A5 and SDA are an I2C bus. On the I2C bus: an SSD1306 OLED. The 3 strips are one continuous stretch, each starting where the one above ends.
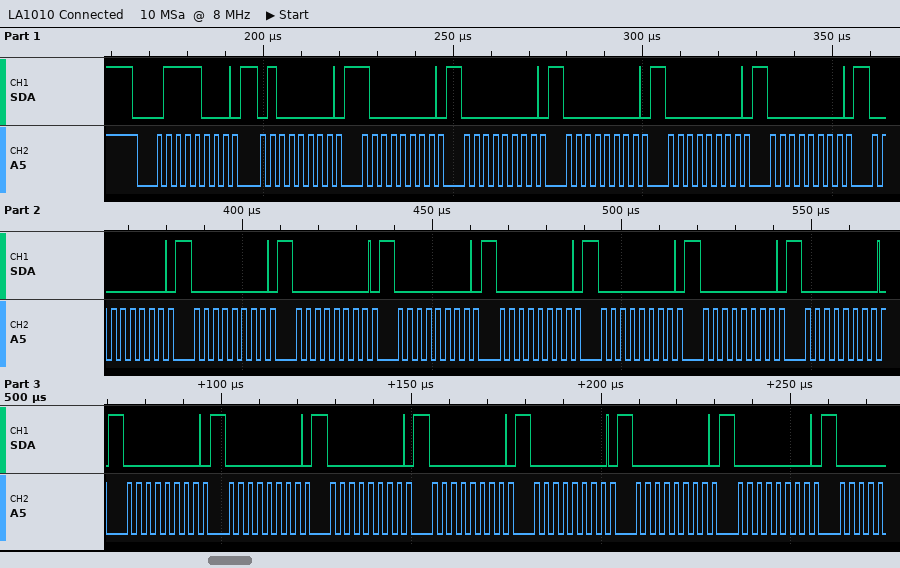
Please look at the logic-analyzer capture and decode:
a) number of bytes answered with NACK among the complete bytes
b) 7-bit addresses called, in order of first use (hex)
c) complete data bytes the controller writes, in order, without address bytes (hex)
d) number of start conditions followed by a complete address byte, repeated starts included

0
0x3C
40 80 00 00 00 00 00 00 00 00 00 00 00 00 00 00 00 00 00 00 00
1
